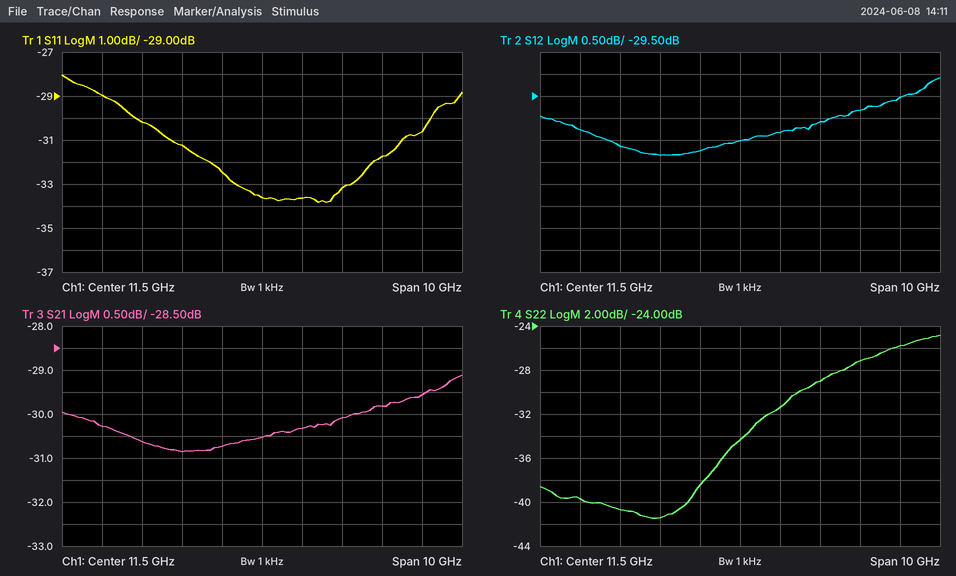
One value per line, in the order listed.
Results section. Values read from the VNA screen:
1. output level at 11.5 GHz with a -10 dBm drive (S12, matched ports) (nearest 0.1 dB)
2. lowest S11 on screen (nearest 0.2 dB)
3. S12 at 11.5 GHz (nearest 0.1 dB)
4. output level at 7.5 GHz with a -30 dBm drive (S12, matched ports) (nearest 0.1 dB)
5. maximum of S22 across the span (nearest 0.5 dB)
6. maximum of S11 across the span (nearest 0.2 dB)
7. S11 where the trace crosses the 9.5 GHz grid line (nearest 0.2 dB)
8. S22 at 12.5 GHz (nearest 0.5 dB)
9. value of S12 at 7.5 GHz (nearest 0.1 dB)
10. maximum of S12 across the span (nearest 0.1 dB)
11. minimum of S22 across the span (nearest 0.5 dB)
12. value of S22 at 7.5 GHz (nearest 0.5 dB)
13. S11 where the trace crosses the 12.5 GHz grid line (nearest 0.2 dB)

-40.5 dBm
-33.8 dB
-30.5 dB
-60.3 dBm
-25.0 dB
-28.0 dB
-31.2 dB
-31.5 dB
-30.3 dB
-29.1 dB
-41.5 dB
-39.5 dB
-33.6 dB
